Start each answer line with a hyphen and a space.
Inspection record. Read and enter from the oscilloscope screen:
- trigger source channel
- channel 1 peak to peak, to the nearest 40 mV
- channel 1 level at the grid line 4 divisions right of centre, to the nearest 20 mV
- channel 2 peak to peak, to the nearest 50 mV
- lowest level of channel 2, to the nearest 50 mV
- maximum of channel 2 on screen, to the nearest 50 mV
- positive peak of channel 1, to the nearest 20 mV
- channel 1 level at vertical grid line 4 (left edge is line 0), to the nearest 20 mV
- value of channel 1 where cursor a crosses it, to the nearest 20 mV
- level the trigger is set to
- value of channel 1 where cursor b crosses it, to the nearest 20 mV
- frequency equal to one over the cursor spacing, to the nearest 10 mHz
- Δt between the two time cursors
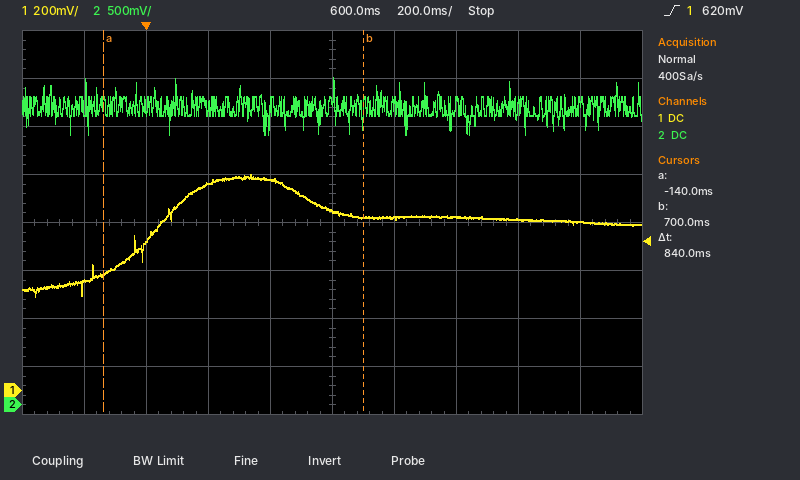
- channel 1
- 520 mV
- 700 mV
- 600 mV
- 2.80 V
- 3.40 V
- 900 mV
- 880 mV
- 480 mV
- 620 mV
- 720 mV
- 1.19 Hz
- 840 ms
